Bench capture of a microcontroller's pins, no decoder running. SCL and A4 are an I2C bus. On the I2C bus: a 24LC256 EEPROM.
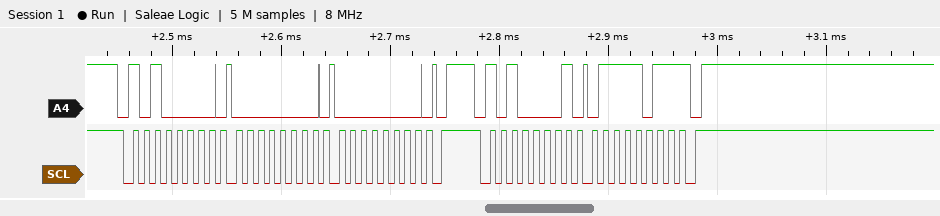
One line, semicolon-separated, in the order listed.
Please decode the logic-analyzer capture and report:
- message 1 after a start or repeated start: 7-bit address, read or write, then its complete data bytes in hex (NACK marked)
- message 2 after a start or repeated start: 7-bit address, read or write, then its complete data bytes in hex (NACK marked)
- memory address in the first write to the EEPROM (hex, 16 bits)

0x50 write: 00 00; 0x50 read: 7B NACK; 0x0000
